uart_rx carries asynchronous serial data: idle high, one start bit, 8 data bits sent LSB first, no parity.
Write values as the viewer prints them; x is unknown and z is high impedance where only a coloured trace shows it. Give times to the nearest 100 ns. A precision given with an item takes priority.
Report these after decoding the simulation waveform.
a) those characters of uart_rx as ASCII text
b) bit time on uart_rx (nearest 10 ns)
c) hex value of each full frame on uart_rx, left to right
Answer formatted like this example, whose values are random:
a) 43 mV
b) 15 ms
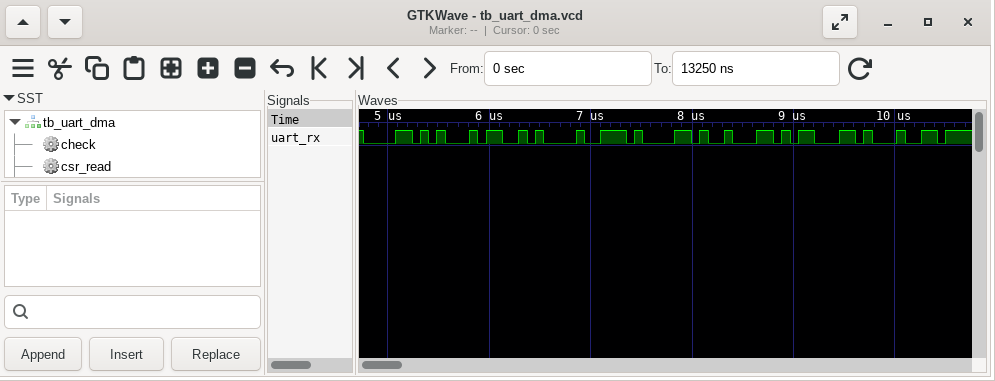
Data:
a) "X4!abcd"
b) 80 ns
c) 58, 34, 21, 61, 62, 63, 64
